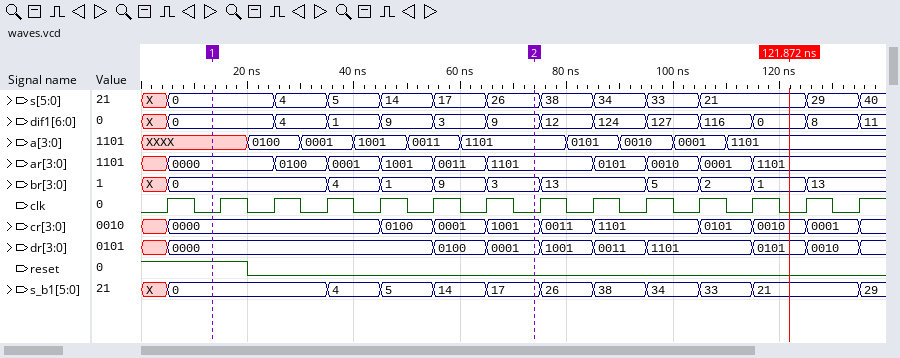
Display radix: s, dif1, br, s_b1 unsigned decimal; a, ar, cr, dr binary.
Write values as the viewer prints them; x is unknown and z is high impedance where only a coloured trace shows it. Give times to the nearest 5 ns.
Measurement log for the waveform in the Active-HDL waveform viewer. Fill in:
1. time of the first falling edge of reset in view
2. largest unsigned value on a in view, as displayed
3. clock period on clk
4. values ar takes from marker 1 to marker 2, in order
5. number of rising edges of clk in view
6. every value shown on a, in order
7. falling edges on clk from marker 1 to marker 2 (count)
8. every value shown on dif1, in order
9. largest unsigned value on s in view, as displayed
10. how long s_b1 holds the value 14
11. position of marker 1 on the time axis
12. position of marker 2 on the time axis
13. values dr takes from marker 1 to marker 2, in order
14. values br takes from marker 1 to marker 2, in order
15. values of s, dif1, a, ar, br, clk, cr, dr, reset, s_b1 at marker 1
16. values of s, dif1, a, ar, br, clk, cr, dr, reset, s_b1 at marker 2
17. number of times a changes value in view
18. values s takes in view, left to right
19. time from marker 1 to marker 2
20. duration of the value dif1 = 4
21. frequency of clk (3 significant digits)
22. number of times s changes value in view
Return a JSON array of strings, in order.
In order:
["20 ns", "1101", "10 ns", "0000, 0100, 0001, 1001, 0011, 1101", "14", "XXXX, 0100, 0001, 1001, 0011, 1101, 0101, 0010, 0001, 1101", "6", "X, 0, 4, 1, 9, 3, 9, 12, 124, 127, 116, 0, 8, 11", "40", "10 ns", "15 ns", "75 ns", "0000, 0100, 0001", "0, 4, 1, 9, 3", "s=0, dif1=0, a=XXXX, ar=0000, br=0, clk=0, cr=0000, dr=0000, reset=1, s_b1=0", "s=26, dif1=9, a=1101, ar=1101, br=3, clk=0, cr=1001, dr=0001, reset=0, s_b1=17", "9", "X, 0, 4, 5, 14, 17, 26, 38, 34, 33, 21, 29, 40", "60 ns", "10 ns", "100 MHz", "12"]
